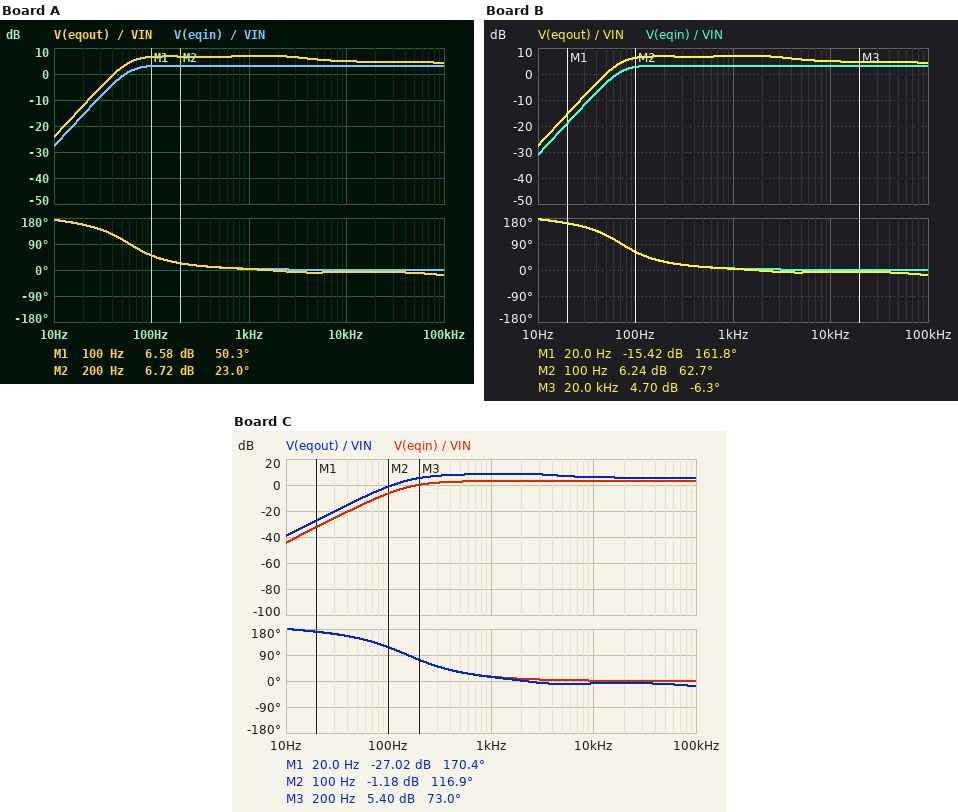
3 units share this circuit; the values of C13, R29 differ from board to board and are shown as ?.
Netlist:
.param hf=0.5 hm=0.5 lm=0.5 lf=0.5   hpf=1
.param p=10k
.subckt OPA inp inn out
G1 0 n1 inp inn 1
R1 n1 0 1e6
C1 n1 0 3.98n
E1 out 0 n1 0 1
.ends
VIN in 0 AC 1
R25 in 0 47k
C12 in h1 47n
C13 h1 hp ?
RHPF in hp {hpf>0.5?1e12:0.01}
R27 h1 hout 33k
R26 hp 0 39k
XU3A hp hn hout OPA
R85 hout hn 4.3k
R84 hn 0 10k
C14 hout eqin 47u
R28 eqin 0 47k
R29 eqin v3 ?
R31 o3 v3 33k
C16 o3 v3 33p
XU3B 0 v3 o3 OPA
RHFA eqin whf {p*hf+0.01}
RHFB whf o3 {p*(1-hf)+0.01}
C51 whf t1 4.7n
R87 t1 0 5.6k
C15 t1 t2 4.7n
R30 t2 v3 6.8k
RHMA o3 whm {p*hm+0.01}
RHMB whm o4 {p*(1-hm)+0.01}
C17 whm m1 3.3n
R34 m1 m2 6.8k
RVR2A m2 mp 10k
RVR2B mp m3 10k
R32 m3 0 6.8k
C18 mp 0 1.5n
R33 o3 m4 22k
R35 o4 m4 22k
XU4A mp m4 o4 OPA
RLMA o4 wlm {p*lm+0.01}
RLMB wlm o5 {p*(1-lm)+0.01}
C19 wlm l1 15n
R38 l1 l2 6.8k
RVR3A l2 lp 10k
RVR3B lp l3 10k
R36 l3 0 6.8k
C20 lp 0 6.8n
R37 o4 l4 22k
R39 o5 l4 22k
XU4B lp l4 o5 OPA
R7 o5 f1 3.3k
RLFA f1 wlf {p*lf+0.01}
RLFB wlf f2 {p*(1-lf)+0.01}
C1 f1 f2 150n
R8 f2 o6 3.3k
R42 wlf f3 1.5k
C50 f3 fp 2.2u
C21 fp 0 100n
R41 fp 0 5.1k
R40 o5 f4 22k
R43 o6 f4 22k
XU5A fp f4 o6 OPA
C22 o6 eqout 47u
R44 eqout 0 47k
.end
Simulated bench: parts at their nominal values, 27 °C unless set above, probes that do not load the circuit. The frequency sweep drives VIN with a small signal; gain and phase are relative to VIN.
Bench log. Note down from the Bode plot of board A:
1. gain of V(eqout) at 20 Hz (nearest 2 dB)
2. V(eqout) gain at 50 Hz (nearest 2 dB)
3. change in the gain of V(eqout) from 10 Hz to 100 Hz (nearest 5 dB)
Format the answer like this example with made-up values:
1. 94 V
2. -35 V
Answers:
1. -12 dB
2. 2 dB
3. 30 dB
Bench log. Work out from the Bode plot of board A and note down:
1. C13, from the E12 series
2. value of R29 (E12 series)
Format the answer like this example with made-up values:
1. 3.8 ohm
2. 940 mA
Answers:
1. 120 nF
2. 22 kΩ
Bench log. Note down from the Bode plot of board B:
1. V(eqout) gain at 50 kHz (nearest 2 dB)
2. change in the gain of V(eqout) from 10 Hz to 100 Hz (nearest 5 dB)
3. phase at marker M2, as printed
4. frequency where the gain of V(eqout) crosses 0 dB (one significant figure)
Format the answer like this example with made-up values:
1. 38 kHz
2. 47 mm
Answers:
1. 4 dB
2. 35 dB
3. 62.7 deg
4. 50 Hz
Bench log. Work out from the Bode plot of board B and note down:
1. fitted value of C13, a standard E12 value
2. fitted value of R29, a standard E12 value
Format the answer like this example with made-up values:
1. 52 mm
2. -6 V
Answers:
1. 82 nF
2. 22 kΩ
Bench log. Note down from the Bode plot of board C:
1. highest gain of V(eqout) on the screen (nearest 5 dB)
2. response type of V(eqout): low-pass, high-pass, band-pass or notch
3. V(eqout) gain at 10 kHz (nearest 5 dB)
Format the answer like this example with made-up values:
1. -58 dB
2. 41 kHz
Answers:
1. 10 dB
2. high-pass
3. 5 dB
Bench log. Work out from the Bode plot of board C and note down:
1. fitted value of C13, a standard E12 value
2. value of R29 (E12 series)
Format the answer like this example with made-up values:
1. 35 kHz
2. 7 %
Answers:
1. 18 nF
2. 18 kΩ
